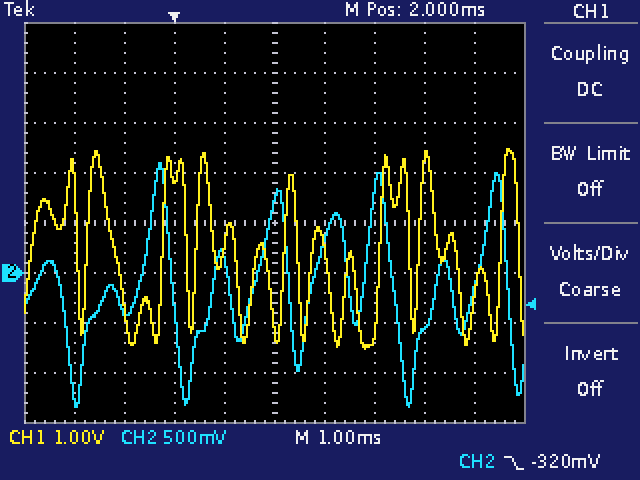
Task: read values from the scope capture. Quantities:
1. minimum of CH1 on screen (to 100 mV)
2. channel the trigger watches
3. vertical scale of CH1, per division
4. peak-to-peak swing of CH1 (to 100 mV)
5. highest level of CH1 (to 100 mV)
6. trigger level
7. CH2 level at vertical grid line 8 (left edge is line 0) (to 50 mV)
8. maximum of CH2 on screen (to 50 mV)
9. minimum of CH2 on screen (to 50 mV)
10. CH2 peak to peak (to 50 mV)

-1.5 V
CH2
1 V
4.0 V
2.5 V
-320 mV
-550 mV
1.10 V
-1.35 V
2.45 V
